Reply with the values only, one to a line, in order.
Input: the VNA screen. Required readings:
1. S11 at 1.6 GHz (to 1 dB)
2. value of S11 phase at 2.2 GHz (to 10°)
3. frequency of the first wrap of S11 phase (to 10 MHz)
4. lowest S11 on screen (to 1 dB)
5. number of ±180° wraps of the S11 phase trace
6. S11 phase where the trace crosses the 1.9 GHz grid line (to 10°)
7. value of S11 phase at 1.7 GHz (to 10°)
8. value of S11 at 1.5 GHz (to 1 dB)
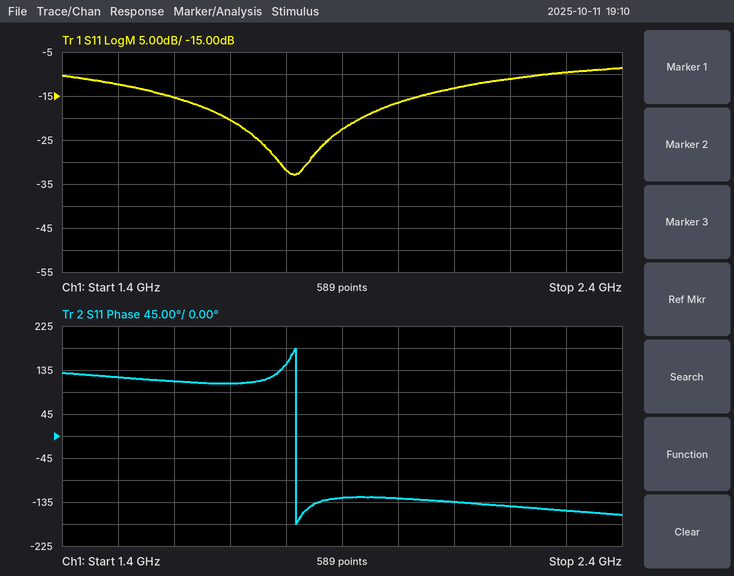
-15 dB
-140°
1.82 GHz
-33 dB
1
-130°
110°
-12 dB
